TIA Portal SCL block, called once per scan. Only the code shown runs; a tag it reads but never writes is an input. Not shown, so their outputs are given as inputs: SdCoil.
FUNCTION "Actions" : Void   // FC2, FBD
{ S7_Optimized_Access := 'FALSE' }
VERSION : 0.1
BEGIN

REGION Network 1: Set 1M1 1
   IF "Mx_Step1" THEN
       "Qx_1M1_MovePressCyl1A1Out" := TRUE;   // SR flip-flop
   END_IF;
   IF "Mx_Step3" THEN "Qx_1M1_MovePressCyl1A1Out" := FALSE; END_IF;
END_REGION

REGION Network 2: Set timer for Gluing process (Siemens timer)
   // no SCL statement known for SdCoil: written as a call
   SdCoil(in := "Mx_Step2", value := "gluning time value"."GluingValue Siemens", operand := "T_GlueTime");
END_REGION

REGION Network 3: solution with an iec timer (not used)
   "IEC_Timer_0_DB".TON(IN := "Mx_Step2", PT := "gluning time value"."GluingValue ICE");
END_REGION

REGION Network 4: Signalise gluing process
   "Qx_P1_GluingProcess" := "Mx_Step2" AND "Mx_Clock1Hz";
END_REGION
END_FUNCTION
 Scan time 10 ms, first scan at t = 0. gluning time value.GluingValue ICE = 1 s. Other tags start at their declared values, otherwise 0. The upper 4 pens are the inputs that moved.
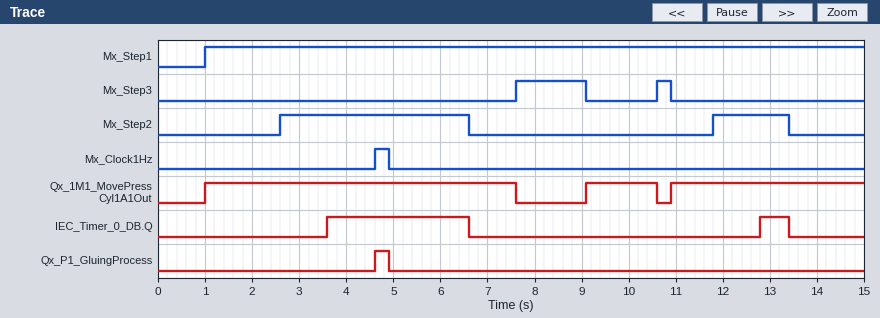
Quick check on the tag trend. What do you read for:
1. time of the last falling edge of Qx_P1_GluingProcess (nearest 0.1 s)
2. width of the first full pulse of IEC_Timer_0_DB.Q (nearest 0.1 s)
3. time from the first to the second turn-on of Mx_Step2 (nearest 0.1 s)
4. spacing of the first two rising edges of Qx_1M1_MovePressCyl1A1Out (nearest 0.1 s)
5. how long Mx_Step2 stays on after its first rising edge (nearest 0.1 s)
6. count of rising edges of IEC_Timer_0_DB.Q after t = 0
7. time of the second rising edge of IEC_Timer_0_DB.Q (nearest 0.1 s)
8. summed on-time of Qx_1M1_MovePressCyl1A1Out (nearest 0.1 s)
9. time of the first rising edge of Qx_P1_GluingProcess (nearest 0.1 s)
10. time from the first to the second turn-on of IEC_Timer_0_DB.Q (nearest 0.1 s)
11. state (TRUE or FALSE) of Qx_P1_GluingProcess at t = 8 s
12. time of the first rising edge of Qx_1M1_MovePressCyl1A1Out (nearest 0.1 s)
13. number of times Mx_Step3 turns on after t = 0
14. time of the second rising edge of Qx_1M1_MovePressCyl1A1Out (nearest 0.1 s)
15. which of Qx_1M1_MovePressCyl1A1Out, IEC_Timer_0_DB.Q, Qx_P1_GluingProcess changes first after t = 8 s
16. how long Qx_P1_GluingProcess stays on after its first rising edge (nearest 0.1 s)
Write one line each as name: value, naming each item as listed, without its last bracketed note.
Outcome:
time of the last falling edge of Qx_P1_GluingProcess: 4.9 s
width of the first full pulse of IEC_Timer_0_DB.Q: 3.0 s
time from the first to the second turn-on of Mx_Step2: 9.2 s
spacing of the first two rising edges of Qx_1M1_MovePressCyl1A1Out: 8.1 s
how long Mx_Step2 stays on after its first rising edge: 4.0 s
count of rising edges of IEC_Timer_0_DB.Q after t = 0: 2
time of the second rising edge of IEC_Timer_0_DB.Q: 12.8 s
summed on-time of Qx_1M1_MovePressCyl1A1Out: 12.2 s
time of the first rising edge of Qx_P1_GluingProcess: 4.6 s
time from the first to the second turn-on of IEC_Timer_0_DB.Q: 9.2 s
state (TRUE or FALSE) of Qx_P1_GluingProcess at t = 8 s: FALSE
time of the first rising edge of Qx_1M1_MovePressCyl1A1Out: 1.0 s
number of times Mx_Step3 turns on after t = 0: 2
time of the second rising edge of Qx_1M1_MovePressCyl1A1Out: 9.1 s
which of Qx_1M1_MovePressCyl1A1Out, IEC_Timer_0_DB.Q, Qx_P1_GluingProcess changes first after t = 8 s: Qx_1M1_MovePressCyl1A1Out
how long Qx_P1_GluingProcess stays on after its first rising edge: 0.3 s
